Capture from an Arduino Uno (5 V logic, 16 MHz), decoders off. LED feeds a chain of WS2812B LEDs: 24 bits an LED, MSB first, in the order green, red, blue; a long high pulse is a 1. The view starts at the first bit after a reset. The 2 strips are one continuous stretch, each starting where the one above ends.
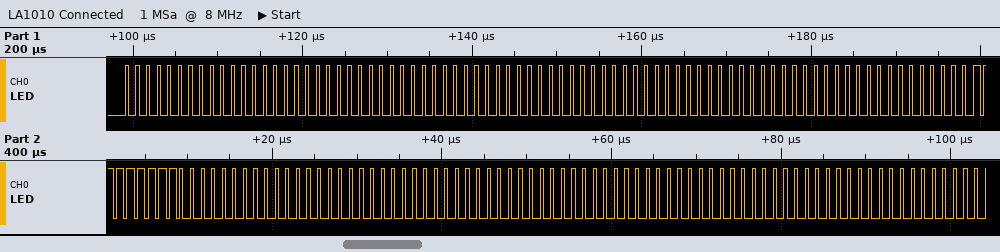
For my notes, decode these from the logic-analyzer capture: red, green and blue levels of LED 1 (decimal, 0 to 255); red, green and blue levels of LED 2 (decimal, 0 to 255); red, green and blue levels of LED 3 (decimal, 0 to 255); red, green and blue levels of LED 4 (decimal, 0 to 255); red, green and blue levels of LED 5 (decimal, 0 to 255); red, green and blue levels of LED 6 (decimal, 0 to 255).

0, 0, 0
0, 0, 0
0, 0, 0
255, 0, 0
0, 0, 0
0, 0, 0
